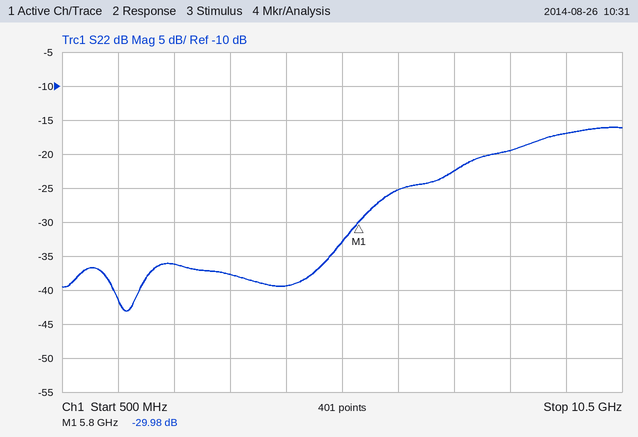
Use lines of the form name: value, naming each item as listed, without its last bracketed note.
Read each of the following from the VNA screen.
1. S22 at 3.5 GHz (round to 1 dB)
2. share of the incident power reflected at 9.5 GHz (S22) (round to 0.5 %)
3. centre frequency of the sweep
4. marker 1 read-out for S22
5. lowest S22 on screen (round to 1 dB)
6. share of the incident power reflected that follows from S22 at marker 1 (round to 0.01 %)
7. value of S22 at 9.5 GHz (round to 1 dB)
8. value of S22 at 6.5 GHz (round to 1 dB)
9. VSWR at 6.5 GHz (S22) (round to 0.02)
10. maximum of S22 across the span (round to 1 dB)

S22 at 3.5 GHz: -38 dB
share of the incident power reflected at 9.5 GHz (S22): 2.0 %
centre frequency of the sweep: 5.5 GHz
marker 1 read-out for S22: -29.98 dB
lowest S22 on screen: -43 dB
share of the incident power reflected that follows from S22 at marker 1: 0.10 %
value of S22 at 9.5 GHz: -17 dB
value of S22 at 6.5 GHz: -25 dB
VSWR at 6.5 GHz (S22): 1.12
maximum of S22 across the span: -16 dB
